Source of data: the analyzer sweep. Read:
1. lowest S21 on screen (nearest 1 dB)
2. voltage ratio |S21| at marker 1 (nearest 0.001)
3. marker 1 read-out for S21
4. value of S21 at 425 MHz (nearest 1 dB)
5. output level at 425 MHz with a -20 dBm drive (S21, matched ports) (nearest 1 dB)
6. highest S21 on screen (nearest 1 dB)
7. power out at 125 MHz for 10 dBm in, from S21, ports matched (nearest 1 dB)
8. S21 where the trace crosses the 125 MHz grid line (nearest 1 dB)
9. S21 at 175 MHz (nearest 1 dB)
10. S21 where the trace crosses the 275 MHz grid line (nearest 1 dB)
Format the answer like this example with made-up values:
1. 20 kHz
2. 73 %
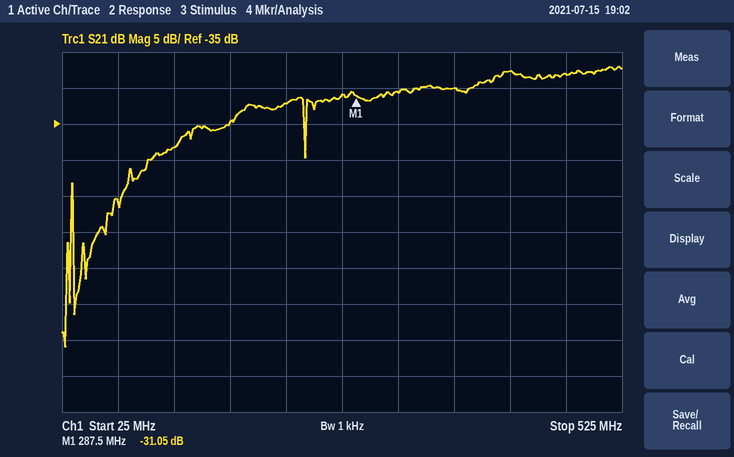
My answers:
1. -66 dB
2. 0.028
3. -31.05 dB
4. -28 dB
5. -48 dBm
6. -27 dB
7. -28 dBm
8. -38 dB
9. -35 dB
10. -31 dB
